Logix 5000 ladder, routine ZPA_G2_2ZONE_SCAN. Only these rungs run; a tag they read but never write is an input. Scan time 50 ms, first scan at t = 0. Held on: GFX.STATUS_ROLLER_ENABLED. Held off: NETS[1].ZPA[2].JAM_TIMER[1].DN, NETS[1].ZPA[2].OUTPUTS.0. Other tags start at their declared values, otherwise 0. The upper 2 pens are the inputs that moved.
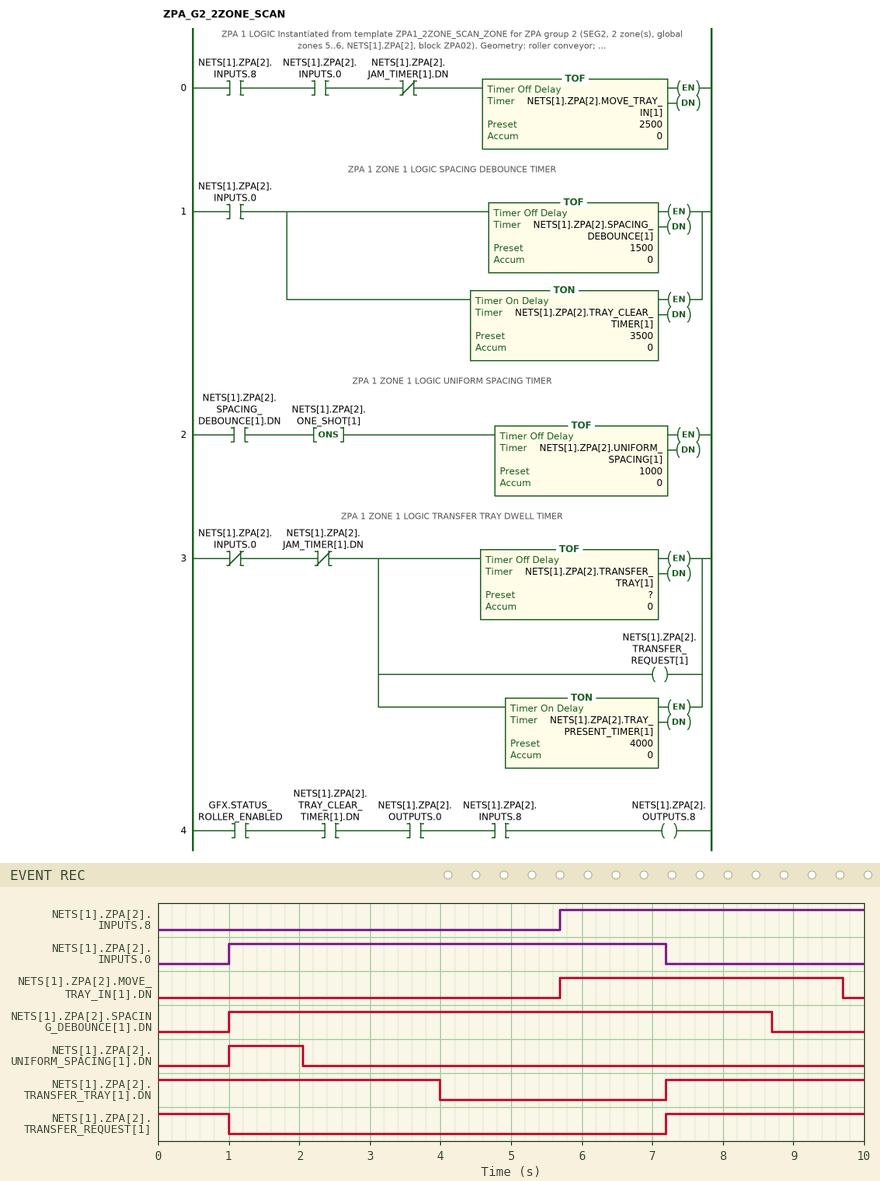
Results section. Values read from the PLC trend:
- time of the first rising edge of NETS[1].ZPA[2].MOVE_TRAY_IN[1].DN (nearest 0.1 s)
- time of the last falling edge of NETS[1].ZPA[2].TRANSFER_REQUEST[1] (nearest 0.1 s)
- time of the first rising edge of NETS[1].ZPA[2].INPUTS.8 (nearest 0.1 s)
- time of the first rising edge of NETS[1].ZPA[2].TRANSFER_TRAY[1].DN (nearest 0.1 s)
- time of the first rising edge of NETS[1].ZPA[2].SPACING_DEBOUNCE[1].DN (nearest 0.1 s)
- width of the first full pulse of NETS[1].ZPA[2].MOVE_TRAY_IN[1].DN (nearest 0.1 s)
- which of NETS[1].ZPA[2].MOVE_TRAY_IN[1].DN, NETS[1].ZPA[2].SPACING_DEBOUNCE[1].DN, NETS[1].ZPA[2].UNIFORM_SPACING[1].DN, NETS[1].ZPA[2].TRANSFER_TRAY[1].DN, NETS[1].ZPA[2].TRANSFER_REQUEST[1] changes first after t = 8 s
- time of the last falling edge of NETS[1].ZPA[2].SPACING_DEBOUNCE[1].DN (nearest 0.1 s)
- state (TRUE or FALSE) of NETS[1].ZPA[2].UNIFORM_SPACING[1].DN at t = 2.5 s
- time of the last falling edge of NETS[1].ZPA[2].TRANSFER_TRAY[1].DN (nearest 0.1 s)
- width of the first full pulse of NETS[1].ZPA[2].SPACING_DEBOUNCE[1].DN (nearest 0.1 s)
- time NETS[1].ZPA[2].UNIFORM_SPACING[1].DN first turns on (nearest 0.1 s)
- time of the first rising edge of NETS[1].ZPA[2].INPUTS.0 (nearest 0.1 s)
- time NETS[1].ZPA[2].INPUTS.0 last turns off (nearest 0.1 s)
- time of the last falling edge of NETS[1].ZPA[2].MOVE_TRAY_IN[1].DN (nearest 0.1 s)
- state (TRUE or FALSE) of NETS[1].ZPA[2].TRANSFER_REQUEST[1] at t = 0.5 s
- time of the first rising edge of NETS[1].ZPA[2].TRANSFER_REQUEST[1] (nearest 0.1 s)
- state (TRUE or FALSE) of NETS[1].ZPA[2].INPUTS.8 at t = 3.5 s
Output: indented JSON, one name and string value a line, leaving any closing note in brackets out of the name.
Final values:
{
  "time of the first rising edge of NETS[1].ZPA[2].MOVE_TRAY_IN[1].DN": "5.7 s",
  "time of the last falling edge of NETS[1].ZPA[2].TRANSFER_REQUEST[1]": "1.0 s",
  "time of the first rising edge of NETS[1].ZPA[2].INPUTS.8": "5.7 s",
  "time of the first rising edge of NETS[1].ZPA[2].TRANSFER_TRAY[1].DN": "7.2 s",
  "time of the first rising edge of NETS[1].ZPA[2].SPACING_DEBOUNCE[1].DN": "1.0 s",
  "width of the first full pulse of NETS[1].ZPA[2].MOVE_TRAY_IN[1].DN": "4.0 s",
  "which of NETS[1].ZPA[2].MOVE_TRAY_IN[1].DN, NETS[1].ZPA[2].SPACING_DEBOUNCE[1].DN, NETS[1].ZPA[2].UNIFORM_SPACING[1].DN, NETS[1].ZPA[2].TRANSFER_TRAY[1].DN, NETS[1].ZPA[2].TRANSFER_REQUEST[1] changes first after t = 8 s": "NETS[1].ZPA[2].SPACING_DEBOUNCE[1].DN",
  "time of the last falling edge of NETS[1].ZPA[2].SPACING_DEBOUNCE[1].DN": "8.7 s",
  "state (TRUE or FALSE) of NETS[1].ZPA[2].UNIFORM_SPACING[1].DN at t = 2.5 s": "FALSE",
  "time of the last falling edge of NETS[1].ZPA[2].TRANSFER_TRAY[1].DN": "4.0 s",
  "width of the first full pulse of NETS[1].ZPA[2].SPACING_DEBOUNCE[1].DN": "7.7 s",
  "time NETS[1].ZPA[2].UNIFORM_SPACING[1].DN first turns on": "1.0 s",
  "time of the first rising edge of NETS[1].ZPA[2].INPUTS.0": "1.0 s",
  "time NETS[1].ZPA[2].INPUTS.0 last turns off": "7.2 s",
  "time of the last falling edge of NETS[1].ZPA[2].MOVE_TRAY_IN[1].DN": "9.7 s",
  "state (TRUE or FALSE) of NETS[1].ZPA[2].TRANSFER_REQUEST[1] at t = 0.5 s": "TRUE",
  "time of the first rising edge of NETS[1].ZPA[2].TRANSFER_REQUEST[1]": "7.2 s",
  "state (TRUE or FALSE) of NETS[1].ZPA[2].INPUTS.8 at t = 3.5 s": "FALSE"
}
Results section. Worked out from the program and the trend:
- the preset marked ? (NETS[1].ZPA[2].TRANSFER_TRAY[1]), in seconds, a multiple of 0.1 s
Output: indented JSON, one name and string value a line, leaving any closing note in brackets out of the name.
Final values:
{
  "the preset marked ? (NETS[1].ZPA[2].TRANSFER_TRAY[1]), in seconds, a multiple of 0.1 s": "3.0 s"
}
